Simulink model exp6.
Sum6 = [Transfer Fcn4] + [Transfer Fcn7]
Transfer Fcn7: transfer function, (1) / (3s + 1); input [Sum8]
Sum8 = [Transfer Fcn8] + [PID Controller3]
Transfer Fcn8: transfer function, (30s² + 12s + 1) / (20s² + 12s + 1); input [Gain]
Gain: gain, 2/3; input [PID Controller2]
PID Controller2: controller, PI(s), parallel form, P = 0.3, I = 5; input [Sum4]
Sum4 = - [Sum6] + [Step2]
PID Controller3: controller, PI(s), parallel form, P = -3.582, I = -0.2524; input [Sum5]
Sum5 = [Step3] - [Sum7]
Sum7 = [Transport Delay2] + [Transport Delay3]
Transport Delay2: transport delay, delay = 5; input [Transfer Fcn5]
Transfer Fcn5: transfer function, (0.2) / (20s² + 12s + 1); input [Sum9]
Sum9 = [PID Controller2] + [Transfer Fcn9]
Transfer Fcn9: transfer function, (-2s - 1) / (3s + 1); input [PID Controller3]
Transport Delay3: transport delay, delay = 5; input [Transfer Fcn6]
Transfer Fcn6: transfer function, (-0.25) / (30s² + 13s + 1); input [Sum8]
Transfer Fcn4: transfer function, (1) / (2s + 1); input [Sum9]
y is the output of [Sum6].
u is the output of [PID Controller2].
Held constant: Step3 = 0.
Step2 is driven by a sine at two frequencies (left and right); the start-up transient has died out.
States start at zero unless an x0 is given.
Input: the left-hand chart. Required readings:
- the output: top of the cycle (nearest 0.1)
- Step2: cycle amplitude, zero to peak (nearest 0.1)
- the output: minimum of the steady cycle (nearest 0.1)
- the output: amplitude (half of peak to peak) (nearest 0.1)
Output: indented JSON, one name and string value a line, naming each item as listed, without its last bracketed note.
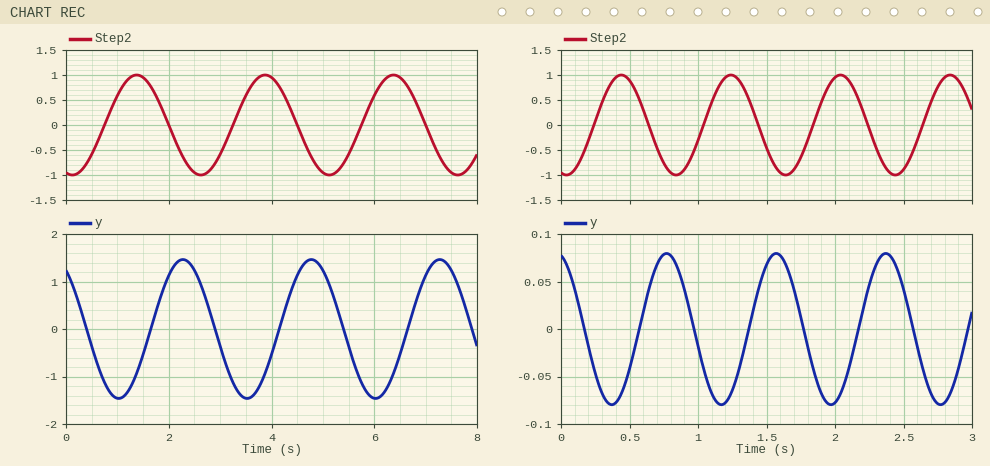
{
  "the output: top of the cycle": "1.5",
  "Step2: cycle amplitude, zero to peak": "1.0",
  "the output: minimum of the steady cycle": "-1.5",
  "the output: amplitude (half of peak to peak)": "1.5"
}
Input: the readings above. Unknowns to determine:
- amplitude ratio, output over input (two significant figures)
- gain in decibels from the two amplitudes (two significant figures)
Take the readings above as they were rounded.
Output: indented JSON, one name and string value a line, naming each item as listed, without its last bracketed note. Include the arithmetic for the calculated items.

{
  "amplitude ratio, output over input": "1.5 / 1 = 1.5",
  "gain in decibels from the two amplitudes": "20 log10(1.5 / 1) = 3.5 dB"
}
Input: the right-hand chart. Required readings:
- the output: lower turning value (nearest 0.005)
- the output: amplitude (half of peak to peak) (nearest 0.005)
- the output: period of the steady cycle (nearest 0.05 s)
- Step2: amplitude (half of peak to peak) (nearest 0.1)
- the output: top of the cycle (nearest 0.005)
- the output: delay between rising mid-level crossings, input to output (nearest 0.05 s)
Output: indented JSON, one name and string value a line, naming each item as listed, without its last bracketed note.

{
  "the output: lower turning value": "-0.080",
  "the output: amplitude (half of peak to peak)": "0.080",
  "the output: period of the steady cycle": "0.80 s",
  "Step2: amplitude (half of peak to peak)": "1.0",
  "the output: top of the cycle": "0.080",
  "the output: delay between rising mid-level crossings, input to output": "0.35 s"
}
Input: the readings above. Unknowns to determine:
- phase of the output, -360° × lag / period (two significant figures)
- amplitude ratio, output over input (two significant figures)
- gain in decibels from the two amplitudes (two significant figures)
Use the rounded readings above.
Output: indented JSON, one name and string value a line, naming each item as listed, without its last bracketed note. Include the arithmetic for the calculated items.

{
  "phase of the output, -360° × lag / period": "-360 × 0.35 / 0.8 = -160°",
  "amplitude ratio, output over input": "0.08 / 1 = 0.080",
  "gain in decibels from the two amplitudes": "20 log10(0.08 / 1) = -22 dB"
}
